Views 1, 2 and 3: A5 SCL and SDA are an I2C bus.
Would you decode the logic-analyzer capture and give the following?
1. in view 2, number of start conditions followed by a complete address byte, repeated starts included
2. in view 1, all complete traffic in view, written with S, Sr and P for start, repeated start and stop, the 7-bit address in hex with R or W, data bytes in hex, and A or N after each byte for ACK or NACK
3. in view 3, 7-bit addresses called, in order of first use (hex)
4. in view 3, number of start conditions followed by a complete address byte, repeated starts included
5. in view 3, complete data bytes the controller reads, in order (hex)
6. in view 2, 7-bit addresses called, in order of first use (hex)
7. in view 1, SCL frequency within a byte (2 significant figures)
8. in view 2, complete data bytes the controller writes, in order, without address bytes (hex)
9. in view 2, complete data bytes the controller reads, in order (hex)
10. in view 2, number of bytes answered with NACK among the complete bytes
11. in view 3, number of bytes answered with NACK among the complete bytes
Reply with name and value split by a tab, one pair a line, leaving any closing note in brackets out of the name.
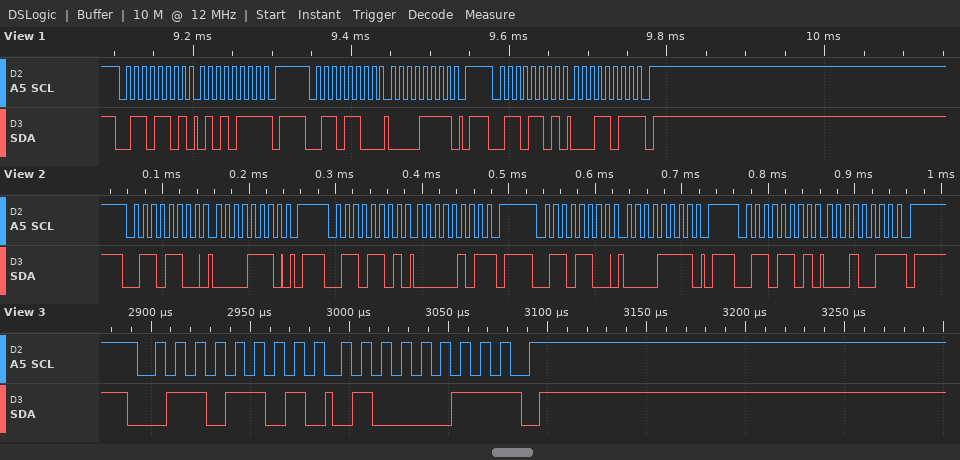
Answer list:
in view 2, number of start conditions followed by a complete address byte, repeated starts included	4
in view 1, all complete traffic in view, written with S, Sr and P for start, repeated start and stop, the 7-bit address in hex with R or W, data bytes in hex, and A or N after each byte for ACK or NACK	S 36R A 57 N P S 36W A 0F A P S 36R A 1B N P
in view 3, 7-bit addresses called, in order of first use	0x36
in view 3, number of start conditions followed by a complete address byte, repeated starts included	1
in view 3, complete data bytes the controller reads, in order	43
in view 2, 7-bit addresses called, in order of first use	0x36
in view 1, SCL frequency within a byte	100 kHz
in view 2, complete data bytes the controller writes, in order, without address bytes	0E 0F
in view 2, complete data bytes the controller reads, in order	05 13
in view 2, number of bytes answered with NACK among the complete bytes	2
in view 3, number of bytes answered with NACK among the complete bytes	1
